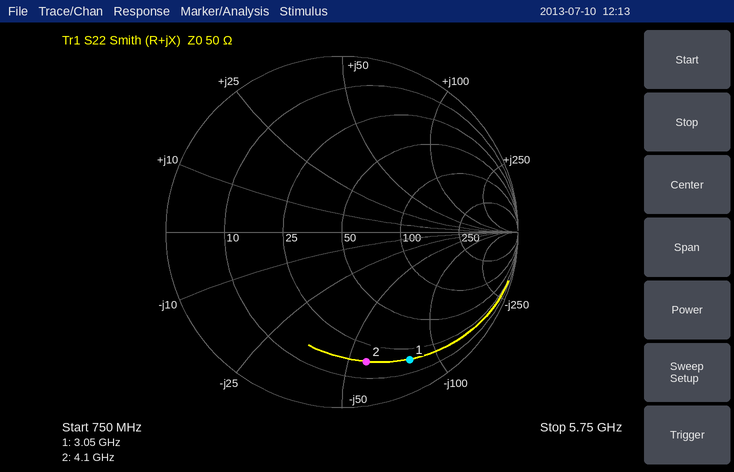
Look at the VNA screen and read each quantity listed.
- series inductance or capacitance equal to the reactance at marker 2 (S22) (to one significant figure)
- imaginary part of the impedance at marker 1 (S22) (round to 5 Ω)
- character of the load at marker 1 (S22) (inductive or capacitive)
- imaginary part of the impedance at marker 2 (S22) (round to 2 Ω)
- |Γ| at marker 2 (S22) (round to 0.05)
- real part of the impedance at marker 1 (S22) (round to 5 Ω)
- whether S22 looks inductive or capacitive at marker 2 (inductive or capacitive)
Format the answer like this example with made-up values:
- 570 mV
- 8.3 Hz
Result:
- 700 fF
- -80 Ω
- capacitive
- -58 Ω
- 0.75
- 20 Ω
- capacitive
